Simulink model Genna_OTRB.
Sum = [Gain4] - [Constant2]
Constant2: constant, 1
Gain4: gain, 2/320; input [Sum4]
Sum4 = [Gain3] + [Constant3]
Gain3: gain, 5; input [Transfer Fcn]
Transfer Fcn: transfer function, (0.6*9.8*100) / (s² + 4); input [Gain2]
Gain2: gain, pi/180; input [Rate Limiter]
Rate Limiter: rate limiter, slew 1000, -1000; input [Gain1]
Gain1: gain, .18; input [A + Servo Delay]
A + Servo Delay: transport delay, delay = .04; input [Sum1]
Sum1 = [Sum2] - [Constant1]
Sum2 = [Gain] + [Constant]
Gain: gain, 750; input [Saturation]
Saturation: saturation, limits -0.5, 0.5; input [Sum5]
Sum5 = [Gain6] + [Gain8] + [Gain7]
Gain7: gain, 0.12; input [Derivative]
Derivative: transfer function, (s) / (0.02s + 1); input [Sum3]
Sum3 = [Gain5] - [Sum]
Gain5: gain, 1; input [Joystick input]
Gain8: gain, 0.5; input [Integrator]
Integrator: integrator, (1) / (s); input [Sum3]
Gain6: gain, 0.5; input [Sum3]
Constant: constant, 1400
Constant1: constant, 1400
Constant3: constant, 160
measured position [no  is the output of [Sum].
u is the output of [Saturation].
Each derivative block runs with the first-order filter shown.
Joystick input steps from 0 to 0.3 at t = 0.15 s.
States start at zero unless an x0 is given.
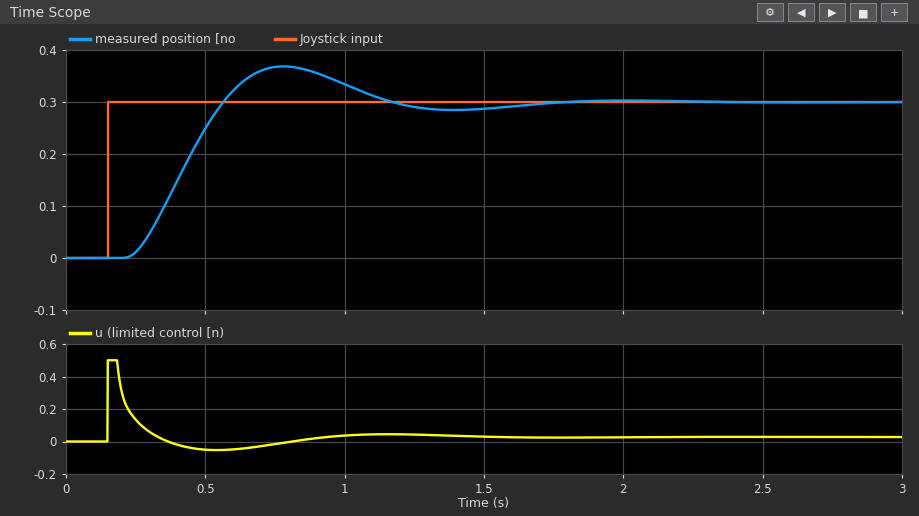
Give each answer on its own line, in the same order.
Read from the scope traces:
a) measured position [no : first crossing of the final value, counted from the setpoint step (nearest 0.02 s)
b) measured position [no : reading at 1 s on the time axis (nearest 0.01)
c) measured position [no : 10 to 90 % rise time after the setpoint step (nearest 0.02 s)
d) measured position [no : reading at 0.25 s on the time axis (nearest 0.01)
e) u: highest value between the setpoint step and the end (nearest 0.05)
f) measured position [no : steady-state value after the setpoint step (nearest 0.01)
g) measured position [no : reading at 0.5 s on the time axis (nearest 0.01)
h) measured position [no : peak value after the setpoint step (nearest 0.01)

0.42 s
0.33
0.24 s
0.01
0.50
0.30
0.25
0.37
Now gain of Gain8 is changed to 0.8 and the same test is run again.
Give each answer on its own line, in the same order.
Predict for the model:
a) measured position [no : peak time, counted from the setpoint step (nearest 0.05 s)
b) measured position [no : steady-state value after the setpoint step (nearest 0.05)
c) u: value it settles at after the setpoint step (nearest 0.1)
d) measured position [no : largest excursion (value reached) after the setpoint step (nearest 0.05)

0.65 s
0.30
0.0
0.40
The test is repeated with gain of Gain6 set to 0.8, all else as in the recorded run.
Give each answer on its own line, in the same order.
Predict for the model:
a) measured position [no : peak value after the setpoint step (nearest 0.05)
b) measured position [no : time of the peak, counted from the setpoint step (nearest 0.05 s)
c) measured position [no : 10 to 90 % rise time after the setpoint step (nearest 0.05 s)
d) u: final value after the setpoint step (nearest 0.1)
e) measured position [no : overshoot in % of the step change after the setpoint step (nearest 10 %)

0.40
0.50 s
0.20 s
0.0
40 %
